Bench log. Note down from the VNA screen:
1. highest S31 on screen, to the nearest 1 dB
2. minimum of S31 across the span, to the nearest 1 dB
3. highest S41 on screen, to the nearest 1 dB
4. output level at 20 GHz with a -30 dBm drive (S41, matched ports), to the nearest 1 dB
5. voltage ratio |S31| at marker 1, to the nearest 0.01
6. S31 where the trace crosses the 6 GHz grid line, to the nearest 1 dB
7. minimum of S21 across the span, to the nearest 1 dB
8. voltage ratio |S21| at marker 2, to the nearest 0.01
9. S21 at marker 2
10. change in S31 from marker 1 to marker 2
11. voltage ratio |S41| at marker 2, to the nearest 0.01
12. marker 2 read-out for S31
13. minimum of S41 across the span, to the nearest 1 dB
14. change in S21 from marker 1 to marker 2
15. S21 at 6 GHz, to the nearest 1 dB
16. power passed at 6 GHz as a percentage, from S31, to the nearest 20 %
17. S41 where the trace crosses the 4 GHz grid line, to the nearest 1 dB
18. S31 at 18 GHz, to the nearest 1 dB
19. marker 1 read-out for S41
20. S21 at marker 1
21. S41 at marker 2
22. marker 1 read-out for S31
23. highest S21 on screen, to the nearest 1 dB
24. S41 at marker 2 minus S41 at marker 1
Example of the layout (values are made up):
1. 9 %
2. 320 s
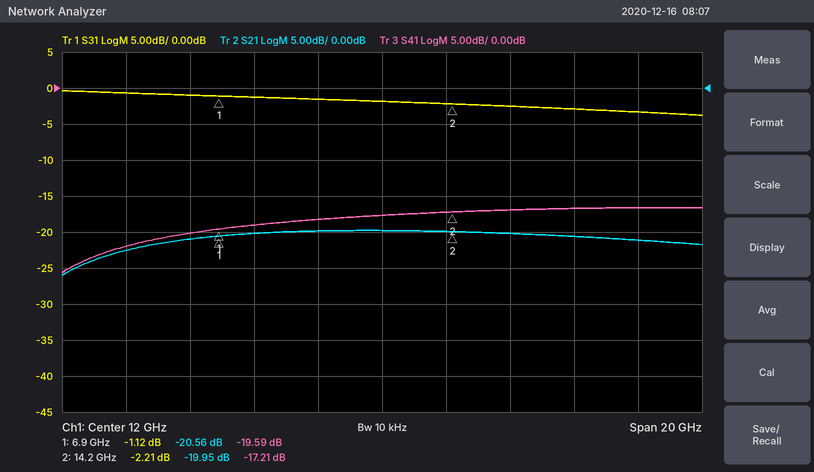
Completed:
1. 0 dB
2. -4 dB
3. -17 dB
4. -47 dBm
5. 0.88
6. -1 dB
7. -26 dB
8. 0.10
9. -19.95 dB
10. -1.09 dB
11. 0.14
12. -2.21 dB
13. -26 dB
14. 0.61 dB
15. -21 dB
16. 80 %
17. -22 dB
18. -3 dB
19. -19.59 dB
20. -20.56 dB
21. -17.21 dB
22. -1.12 dB
23. -20 dB
24. 2.38 dB
